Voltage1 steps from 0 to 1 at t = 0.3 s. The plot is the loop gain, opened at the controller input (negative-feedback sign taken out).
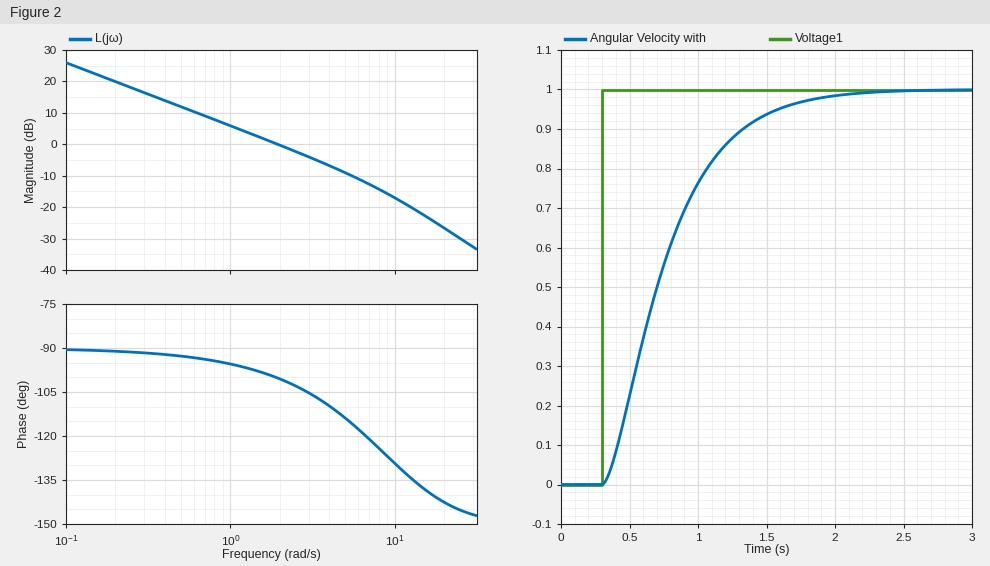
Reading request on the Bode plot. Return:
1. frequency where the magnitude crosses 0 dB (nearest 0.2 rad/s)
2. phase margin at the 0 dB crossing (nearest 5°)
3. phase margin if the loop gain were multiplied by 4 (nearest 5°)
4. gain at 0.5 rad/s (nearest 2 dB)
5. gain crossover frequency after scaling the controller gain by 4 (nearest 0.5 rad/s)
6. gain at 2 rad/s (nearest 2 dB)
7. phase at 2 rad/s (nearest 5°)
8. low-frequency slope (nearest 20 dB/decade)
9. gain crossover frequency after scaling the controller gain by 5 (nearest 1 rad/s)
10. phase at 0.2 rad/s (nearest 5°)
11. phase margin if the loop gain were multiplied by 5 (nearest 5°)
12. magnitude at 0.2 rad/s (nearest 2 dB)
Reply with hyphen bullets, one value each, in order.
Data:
- 2.0 rad/s
- 80°
- 60°
- 12 dB
- 6.5 rad/s
- 0 dB
- -100°
- -20 dB/decade
- 8 rad/s
- -90°
- 55°
- 20 dB
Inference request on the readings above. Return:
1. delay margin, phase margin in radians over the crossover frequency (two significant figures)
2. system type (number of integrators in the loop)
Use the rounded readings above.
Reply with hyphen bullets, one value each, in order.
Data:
- 0.70 s
- 1
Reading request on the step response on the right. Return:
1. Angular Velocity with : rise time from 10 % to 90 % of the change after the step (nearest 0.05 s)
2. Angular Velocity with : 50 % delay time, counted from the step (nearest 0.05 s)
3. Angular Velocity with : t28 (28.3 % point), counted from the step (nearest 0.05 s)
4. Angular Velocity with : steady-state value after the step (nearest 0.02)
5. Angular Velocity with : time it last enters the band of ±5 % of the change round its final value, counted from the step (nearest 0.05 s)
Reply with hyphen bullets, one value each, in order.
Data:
- 0.90 s
- 0.40 s
- 0.25 s
- 1.00
- 1.30 s
